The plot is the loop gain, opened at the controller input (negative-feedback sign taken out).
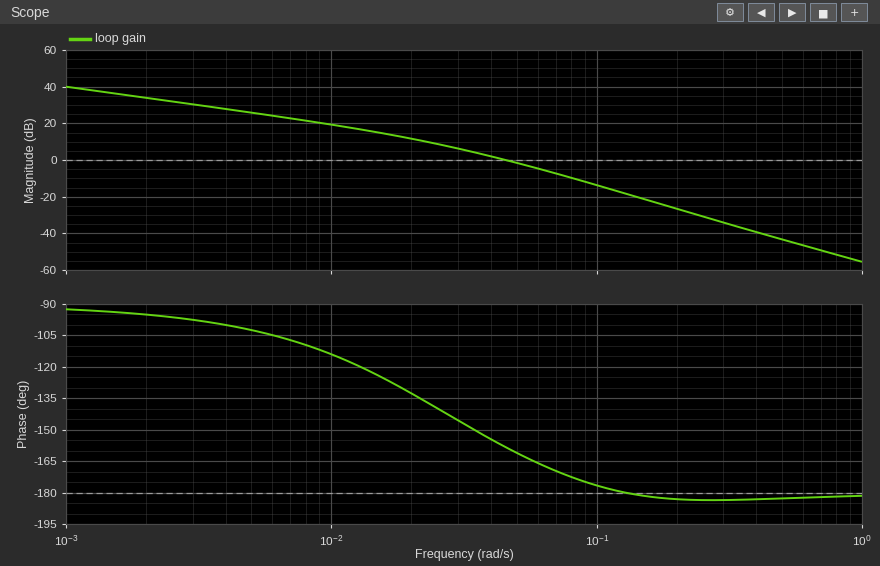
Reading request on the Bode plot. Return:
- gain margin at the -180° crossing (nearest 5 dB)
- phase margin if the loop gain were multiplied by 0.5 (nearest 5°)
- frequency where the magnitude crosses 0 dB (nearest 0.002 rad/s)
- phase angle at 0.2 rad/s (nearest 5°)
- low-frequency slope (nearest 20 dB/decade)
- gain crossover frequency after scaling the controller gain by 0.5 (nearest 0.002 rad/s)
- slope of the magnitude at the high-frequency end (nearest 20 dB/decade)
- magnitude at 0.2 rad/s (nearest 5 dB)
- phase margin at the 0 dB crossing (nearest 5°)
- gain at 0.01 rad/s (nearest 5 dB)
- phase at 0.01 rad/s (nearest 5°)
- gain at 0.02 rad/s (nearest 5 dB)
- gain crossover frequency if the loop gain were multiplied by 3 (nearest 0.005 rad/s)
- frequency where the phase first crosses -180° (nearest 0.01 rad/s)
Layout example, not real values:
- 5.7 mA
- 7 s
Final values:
- 20 dB
- 35°
- 0.046 rad/s
- -185°
- -20 dB/decade
- 0.030 rad/s
- -40 dB/decade
- -25 dB
- 20°
- 20 dB
- -115°
- 10 dB
- 0.080 rad/s
- 0.13 rad/s
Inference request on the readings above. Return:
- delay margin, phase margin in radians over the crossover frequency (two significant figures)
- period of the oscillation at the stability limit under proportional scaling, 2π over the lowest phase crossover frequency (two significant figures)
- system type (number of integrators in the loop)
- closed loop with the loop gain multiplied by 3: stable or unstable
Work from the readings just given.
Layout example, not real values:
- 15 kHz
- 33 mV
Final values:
- 7.6 s
- 48 s
- 1
- stable
